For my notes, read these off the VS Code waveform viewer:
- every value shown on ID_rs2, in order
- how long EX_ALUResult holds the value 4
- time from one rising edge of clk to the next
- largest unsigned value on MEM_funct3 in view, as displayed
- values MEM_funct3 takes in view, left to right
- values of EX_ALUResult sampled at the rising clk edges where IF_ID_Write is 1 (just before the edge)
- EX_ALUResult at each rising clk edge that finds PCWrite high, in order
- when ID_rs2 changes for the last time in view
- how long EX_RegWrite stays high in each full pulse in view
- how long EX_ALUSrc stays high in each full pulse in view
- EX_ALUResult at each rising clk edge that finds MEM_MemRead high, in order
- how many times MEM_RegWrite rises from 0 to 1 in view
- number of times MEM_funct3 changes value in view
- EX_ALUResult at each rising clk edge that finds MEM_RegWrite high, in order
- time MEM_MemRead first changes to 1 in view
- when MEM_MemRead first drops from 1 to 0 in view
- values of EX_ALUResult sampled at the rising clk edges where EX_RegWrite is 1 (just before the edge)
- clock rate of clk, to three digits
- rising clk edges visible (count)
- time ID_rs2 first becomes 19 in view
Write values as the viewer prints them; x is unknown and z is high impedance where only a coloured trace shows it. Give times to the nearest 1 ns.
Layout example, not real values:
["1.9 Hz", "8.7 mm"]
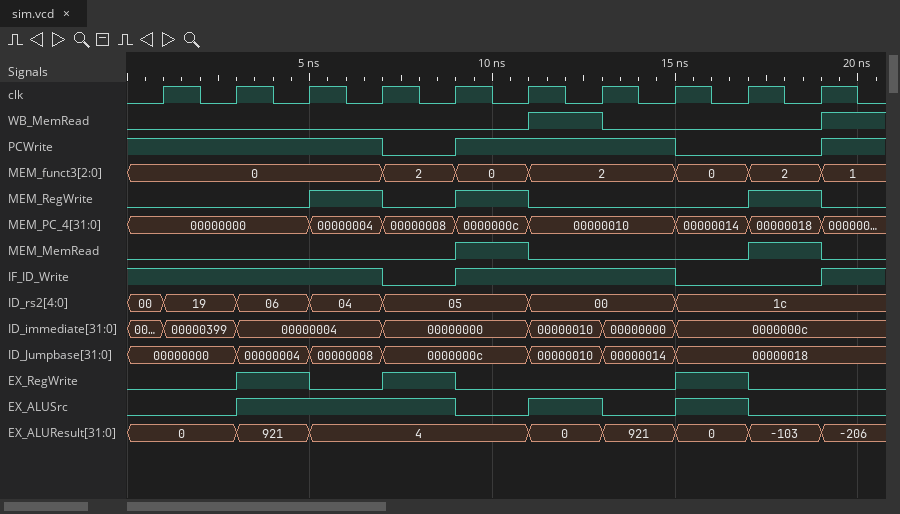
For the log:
["00, 19, 06, 04, 05, 00, 1c", "6 ns", "2 ns", "2", "0, 2, 0, 2, 0, 2, 1", "0, 0, 921, 4, 4, 0, 921", "0, 0, 921, 4, 4, 0, 921", "15 ns", "2 ns, 2 ns, 2 ns", "6 ns, 2 ns, 2 ns", "4, -103", "3", "6", "4, 4, -103", "9 ns", "11 ns", "921, 4, 0", "500 MHz", "10", "1 ns"]
